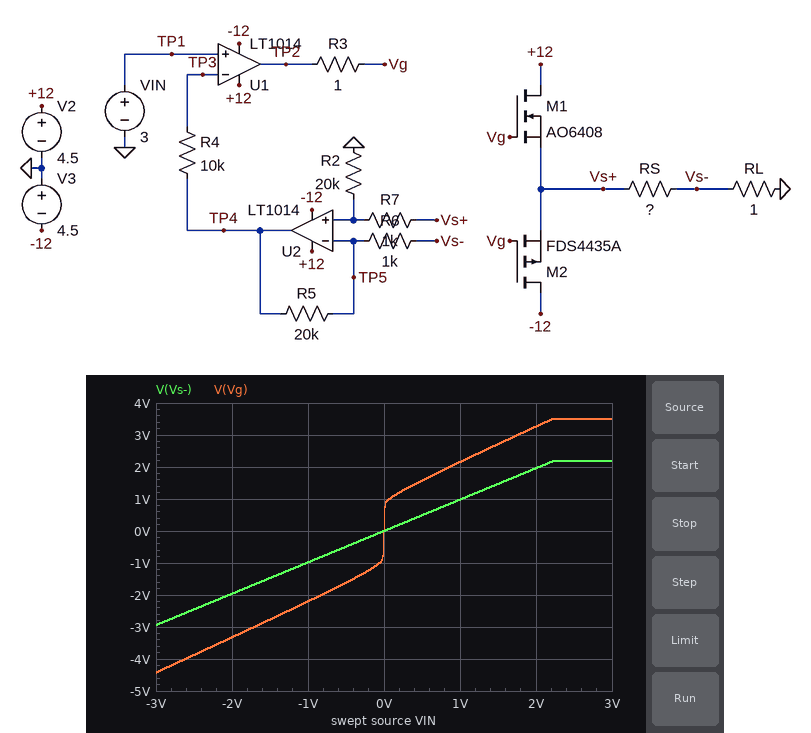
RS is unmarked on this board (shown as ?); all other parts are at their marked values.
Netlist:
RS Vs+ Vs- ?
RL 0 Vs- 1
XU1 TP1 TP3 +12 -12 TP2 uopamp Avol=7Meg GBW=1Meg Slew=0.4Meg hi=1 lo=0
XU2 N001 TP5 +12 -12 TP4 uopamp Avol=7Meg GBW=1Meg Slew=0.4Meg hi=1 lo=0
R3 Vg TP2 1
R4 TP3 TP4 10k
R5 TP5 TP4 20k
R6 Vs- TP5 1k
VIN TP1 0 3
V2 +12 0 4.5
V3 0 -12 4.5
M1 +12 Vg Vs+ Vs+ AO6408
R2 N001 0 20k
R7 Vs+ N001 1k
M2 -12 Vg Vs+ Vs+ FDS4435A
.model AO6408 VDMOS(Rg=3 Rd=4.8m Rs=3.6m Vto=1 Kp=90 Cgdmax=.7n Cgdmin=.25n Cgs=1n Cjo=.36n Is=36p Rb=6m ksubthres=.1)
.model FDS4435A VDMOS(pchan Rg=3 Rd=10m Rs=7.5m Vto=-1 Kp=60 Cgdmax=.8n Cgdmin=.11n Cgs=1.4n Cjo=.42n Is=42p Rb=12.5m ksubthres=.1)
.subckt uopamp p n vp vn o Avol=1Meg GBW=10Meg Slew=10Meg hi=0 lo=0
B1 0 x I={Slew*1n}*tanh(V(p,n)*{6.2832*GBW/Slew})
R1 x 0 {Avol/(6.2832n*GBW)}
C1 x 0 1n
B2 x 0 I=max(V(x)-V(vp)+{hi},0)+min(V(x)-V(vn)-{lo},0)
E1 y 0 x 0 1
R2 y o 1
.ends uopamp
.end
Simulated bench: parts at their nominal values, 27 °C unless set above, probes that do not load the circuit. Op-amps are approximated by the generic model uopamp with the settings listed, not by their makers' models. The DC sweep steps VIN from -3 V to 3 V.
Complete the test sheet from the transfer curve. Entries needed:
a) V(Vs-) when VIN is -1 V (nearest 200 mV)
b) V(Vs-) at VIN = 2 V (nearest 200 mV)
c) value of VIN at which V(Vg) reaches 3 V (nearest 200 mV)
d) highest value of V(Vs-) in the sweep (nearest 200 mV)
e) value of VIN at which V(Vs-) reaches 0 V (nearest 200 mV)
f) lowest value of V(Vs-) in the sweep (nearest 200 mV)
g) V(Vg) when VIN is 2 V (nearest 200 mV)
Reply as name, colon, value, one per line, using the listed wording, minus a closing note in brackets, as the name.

V(Vs-) when VIN is -1 V: -1.0 V
V(Vs-) at VIN = 2 V: 2.0 V
value of VIN at which V(Vg) reaches 3 V: 1.8 V
highest value of V(Vs-) in the sweep: 2.2 V
value of VIN at which V(Vs-) reaches 0 V: 0 V
lowest value of V(Vs-) in the sweep: -3.0 V
V(Vg) when VIN is 2 V: 3.2 V
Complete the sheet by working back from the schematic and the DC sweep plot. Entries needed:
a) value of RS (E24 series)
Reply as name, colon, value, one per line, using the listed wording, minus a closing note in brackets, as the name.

value of RS: 0.051 Ω
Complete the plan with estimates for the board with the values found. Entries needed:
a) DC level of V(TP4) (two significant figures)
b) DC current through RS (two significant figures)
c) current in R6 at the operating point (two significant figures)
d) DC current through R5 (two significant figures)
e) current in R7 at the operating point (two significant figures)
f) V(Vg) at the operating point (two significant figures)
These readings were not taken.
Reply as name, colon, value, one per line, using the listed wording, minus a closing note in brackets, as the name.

DC level of V(TP4): 2.2 V
DC current through RS: 2.2 A
current in R6 at the operating point: 2.1 µA
DC current through R5: 2.1 µA
current in R7 at the operating point: 110 µA
V(Vg) at the operating point: 3.5 V
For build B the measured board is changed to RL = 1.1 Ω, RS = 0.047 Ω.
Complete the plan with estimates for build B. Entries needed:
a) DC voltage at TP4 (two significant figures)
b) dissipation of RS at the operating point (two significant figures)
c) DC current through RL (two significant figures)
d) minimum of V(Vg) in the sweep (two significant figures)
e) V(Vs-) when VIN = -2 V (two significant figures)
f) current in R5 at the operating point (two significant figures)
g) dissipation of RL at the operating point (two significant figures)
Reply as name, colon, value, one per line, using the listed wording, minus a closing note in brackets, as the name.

DC voltage at TP4: 1.9 V
dissipation of RS at the operating point: 190 mW
DC current through RL: 2.0 A
minimum of V(Vg) in the sweep: -4.5 V
V(Vs-) when VIN = -2 V: -2.3 V
current in R5 at the operating point: 15 µA
dissipation of RL at the operating point: 4.4 W
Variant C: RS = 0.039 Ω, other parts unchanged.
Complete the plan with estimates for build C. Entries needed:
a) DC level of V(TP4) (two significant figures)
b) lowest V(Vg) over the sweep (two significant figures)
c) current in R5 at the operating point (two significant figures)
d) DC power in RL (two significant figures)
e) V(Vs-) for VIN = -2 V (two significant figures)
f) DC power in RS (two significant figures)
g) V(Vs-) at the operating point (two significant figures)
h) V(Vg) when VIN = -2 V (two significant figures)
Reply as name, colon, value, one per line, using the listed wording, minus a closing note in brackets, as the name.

DC level of V(TP4): 1.7 V
lowest V(Vg) over the sweep: -4.5 V
current in R5 at the operating point: 23 µA
DC power in RL: 4.8 W
V(Vs-) for VIN = -2 V: -2.6 V
DC power in RS: 190 mW
V(Vs-) at the operating point: 2.2 V
V(Vg) when VIN = -2 V: -4.0 V
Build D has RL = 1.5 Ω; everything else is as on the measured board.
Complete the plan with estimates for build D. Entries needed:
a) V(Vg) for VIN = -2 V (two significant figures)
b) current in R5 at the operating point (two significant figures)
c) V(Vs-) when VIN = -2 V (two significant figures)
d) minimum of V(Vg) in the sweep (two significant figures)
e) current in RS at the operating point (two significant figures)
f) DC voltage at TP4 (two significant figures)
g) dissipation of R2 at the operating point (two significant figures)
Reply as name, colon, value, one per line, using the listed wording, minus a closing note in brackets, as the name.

V(Vg) for VIN = -2 V: -4.3 V
current in R5 at the operating point: 34 µA
V(Vs-) when VIN = -2 V: -2.9 V
minimum of V(Vg) in the sweep: -4.5 V
current in RS at the operating point: 1.5 A
DC voltage at TP4: 1.5 V
dissipation of R2 at the operating point: 250 µW
